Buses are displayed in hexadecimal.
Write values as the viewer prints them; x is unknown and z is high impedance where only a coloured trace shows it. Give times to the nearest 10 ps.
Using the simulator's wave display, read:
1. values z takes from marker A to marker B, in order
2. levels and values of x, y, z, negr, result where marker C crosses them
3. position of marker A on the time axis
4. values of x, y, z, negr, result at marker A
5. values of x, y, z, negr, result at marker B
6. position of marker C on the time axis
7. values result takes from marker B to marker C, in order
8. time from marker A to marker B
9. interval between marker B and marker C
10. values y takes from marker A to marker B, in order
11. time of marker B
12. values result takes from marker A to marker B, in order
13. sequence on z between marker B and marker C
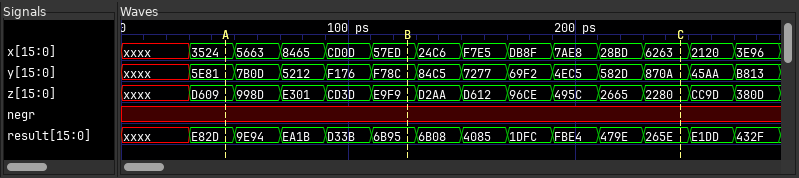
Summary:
D609, 998D, E301, CD3D, E9F9
x=6263, y=870A, z=2280, negr=x, result=265E
50 ps
x=3524, y=5E81, z=D609, negr=x, result=E82D
x=57ED, y=F78C, z=E9F9, negr=x, result=6B95
250 ps
6B95, 6B08, 4085, 1DFC, FBE4, 479E, 265E
80 ps
120 ps
5E81, 7B0D, 5212, F176, F78C
130 ps
E82D, 9E94, EA1B, D33B, 6B95
E9F9, D2AA, D612, 96CE, 495C, 2665, 2280
